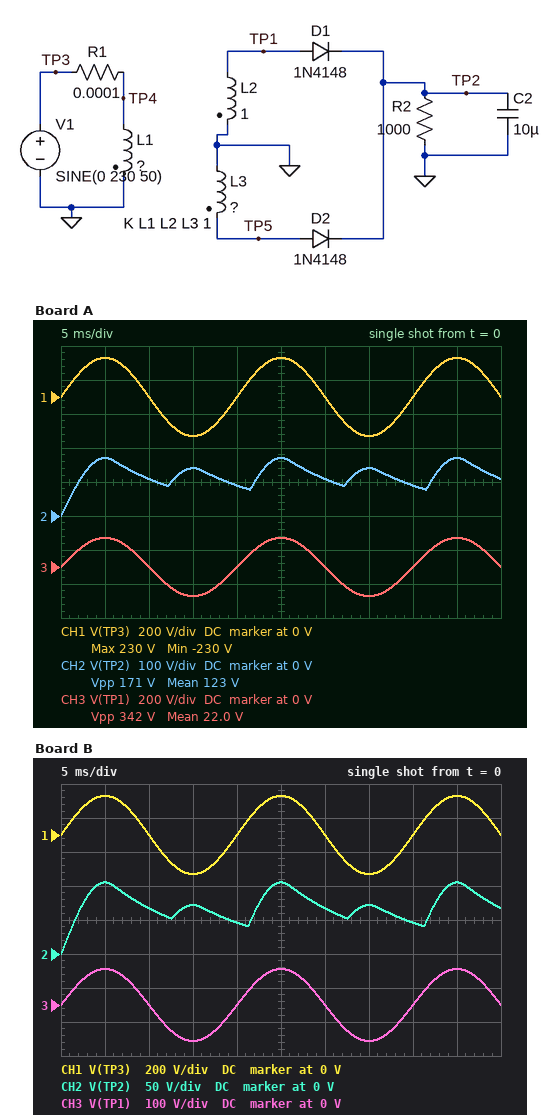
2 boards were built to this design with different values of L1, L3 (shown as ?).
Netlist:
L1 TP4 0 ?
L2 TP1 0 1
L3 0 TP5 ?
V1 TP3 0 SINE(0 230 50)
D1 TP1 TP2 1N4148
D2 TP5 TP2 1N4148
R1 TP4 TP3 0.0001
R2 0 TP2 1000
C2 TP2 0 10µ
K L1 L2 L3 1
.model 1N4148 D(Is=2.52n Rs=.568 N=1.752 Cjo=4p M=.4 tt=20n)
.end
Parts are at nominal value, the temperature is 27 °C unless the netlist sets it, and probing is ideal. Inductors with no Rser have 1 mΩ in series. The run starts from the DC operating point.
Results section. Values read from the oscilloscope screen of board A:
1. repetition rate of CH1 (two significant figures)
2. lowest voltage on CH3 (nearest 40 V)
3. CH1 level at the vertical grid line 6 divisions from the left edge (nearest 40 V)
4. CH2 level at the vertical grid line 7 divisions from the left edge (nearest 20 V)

50 Hz
-160 V
0 V
140 V
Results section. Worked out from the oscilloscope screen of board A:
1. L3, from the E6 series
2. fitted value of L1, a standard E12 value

680 mH
1.8 H
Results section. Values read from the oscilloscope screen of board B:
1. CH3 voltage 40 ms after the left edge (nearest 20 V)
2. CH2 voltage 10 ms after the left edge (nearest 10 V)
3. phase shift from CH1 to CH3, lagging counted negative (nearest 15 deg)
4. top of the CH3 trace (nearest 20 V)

0 V
70 V
0 deg
100 V
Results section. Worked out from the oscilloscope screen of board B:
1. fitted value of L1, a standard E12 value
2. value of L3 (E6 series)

4.7 H
470 mH
